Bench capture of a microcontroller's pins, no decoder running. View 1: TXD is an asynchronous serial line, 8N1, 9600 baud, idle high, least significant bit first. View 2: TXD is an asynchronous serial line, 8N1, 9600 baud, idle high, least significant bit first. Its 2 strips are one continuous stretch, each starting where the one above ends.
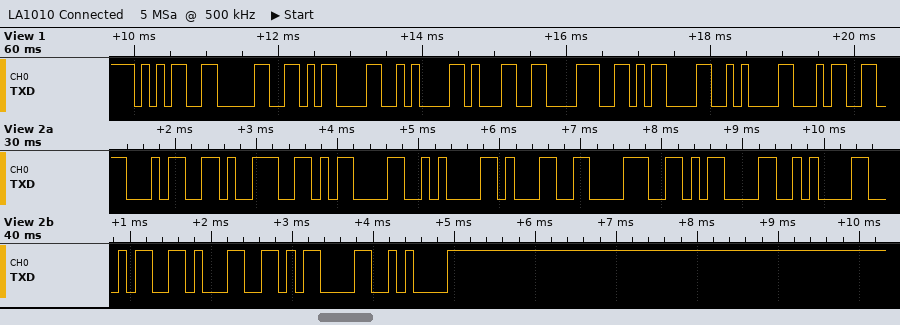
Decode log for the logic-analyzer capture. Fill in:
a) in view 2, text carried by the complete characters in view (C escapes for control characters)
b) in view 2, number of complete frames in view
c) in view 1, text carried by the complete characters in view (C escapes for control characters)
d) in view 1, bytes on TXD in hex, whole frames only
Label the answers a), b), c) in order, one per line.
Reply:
a) "49\r\n18\r\n41\r\n"
b) 12
c) "50\r\n18\r\n4"
d) 0x35 0x30 0x0D 0x0A 0x31 0x38 0x0D 0x0A 0x34
